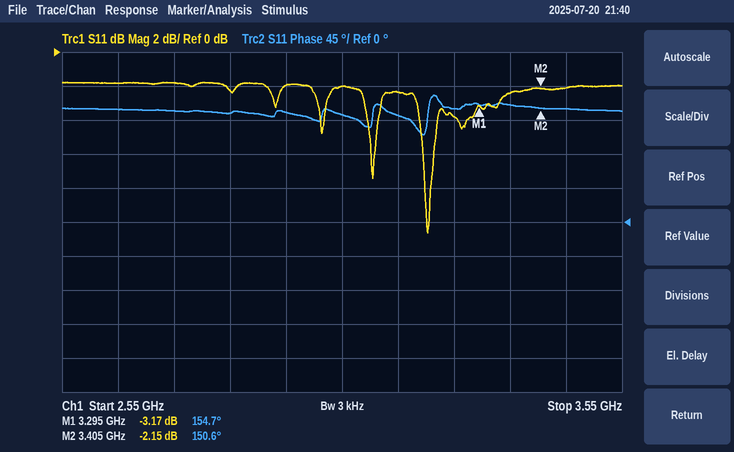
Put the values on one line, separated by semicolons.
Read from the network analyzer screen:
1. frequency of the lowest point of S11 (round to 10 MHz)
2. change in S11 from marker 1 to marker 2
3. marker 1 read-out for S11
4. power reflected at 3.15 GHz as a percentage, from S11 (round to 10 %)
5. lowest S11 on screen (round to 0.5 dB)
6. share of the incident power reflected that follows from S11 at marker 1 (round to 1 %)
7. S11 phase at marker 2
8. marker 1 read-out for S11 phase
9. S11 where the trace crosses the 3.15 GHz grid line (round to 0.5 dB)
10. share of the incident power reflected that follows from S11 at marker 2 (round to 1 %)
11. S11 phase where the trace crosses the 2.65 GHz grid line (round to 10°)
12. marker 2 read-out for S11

3.20 GHz; 1.02 dB; -3.17 dB; 60 %; -10.5 dB; 48 %; 150.6°; 154.7°; -2.5 dB; 61 %; 150°; -2.15 dB
